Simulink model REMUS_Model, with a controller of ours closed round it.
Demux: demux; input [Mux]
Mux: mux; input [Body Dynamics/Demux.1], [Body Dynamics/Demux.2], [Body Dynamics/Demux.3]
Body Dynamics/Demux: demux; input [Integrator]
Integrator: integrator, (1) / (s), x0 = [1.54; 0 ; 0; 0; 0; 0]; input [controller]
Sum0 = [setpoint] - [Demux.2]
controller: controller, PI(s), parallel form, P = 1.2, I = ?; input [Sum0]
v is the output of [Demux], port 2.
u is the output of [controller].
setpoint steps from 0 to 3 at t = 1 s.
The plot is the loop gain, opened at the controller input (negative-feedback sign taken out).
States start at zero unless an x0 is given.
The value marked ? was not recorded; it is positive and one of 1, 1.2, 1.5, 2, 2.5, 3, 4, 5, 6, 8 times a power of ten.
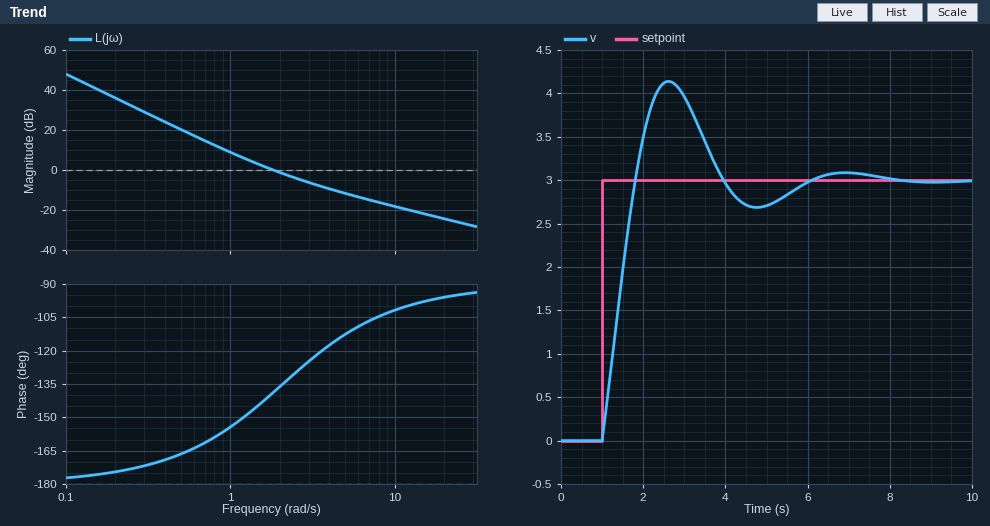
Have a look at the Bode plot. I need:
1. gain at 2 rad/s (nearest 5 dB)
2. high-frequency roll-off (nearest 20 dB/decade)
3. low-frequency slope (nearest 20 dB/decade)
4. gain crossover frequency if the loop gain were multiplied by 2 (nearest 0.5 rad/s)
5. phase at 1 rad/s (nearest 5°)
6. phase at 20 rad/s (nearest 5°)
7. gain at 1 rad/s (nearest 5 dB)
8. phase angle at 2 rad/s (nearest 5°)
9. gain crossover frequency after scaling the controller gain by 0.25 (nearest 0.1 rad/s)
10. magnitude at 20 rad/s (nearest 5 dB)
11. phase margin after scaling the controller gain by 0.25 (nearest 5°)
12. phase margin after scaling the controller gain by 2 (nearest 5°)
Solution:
0 dB
-20 dB/decade
-40 dB/decade
3.0 rad/s
-155°
-95°
10 dB
-135°
0.8 rad/s
-25 dB
20°
55°
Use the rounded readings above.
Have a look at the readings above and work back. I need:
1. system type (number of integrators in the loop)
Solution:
2
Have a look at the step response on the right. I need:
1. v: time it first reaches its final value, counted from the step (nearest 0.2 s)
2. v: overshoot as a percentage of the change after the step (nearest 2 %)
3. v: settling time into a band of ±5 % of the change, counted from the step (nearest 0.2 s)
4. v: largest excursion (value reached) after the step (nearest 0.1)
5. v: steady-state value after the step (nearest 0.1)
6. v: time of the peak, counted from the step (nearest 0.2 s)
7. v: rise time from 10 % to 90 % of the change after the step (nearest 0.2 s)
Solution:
0.8 s
38 %
4.6 s
4.1
3.0
1.6 s
0.6 s
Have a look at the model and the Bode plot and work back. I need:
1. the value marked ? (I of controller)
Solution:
2.5
